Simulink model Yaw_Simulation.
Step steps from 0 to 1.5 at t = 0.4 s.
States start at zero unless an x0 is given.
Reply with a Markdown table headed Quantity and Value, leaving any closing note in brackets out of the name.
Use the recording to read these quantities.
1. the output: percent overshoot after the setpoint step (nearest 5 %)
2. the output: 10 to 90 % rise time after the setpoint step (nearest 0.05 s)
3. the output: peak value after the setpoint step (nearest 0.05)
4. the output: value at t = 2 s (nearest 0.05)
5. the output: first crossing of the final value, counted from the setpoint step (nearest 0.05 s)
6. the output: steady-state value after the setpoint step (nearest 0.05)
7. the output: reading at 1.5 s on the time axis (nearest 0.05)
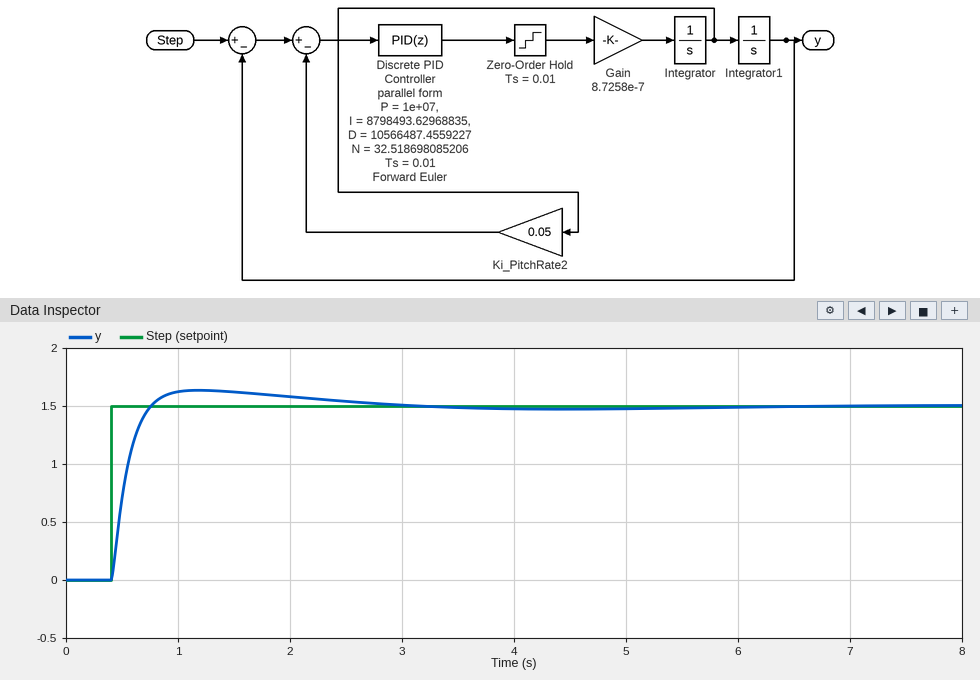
| Quantity | Value |
|---|---|
| the output: percent overshoot after the setpoint step | 10 % |
| the output: 10 to 90 % rise time after the setpoint step | 0.25 s |
| the output: peak value after the setpoint step | 1.65 |
| the output: value at t = 2 s | 1.60 |
| the output: first crossing of the final value, counted from the setpoint step | 0.35 s |
| the output: steady-state value after the setpoint step | 1.50 |
| the output: reading at 1.5 s on the time axis | 1.60 |
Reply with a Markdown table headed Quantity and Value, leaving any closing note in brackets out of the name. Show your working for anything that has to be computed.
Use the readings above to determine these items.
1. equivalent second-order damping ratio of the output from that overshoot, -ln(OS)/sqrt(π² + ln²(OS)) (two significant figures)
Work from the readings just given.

| Quantity | Value |
|---|---|
| equivalent second-order damping ratio of the output from that overshoot, -ln(OS)/sqrt(π² + ln²(OS)) | ln(0.1) = -2.303; 2.303 / sqrt(9.870 + 5.302) = 0.59 |
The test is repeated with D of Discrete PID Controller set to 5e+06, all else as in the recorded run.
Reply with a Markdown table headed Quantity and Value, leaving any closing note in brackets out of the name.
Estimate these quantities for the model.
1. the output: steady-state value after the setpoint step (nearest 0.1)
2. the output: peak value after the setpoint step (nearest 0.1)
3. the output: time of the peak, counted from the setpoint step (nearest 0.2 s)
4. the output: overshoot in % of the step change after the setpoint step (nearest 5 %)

| Quantity | Value |
|---|---|
| the output: steady-state value after the setpoint step | 1.5 |
| the output: peak value after the setpoint step | 1.9 |
| the output: time of the peak, counted from the setpoint step | 0.8 s |
| the output: overshoot in % of the step change after the setpoint step | 25 % |
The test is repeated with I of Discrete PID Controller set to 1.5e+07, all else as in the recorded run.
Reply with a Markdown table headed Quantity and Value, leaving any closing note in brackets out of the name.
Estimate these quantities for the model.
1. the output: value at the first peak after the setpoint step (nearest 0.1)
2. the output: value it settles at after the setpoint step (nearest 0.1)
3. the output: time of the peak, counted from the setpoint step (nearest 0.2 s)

| Quantity | Value |
|---|---|
| the output: value at the first peak after the setpoint step | 1.7 |
| the output: value it settles at after the setpoint step | 1.5 |
| the output: time of the peak, counted from the setpoint step | 0.8 s |
